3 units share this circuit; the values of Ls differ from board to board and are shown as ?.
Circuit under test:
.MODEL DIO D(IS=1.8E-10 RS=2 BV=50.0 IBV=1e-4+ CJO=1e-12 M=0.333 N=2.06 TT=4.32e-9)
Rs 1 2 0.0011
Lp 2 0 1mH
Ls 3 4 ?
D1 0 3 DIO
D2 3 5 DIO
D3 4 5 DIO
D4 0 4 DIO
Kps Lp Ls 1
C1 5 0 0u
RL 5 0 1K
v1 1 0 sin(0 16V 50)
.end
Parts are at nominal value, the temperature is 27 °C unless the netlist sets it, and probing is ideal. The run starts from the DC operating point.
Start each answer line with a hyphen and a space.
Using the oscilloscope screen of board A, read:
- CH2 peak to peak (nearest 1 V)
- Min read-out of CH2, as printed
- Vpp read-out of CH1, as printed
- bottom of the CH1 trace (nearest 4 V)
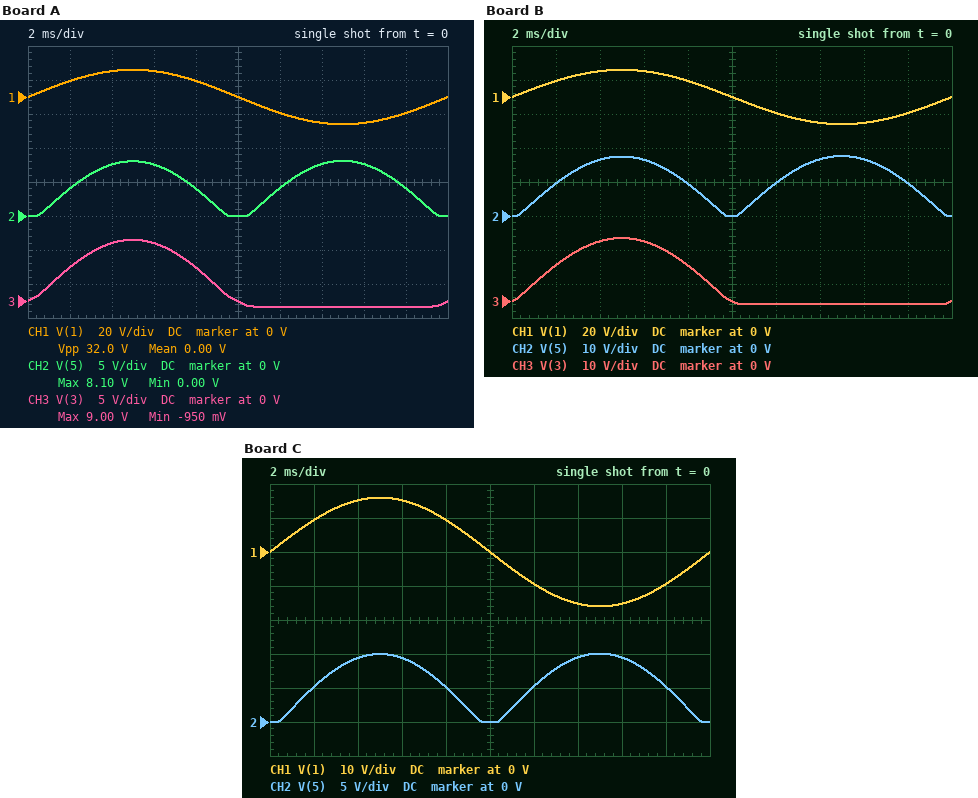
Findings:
- 8 V
- 0.00 V
- 32.0 V
- -16 V
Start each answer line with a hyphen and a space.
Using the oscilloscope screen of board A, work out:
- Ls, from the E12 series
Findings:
- 390 µH
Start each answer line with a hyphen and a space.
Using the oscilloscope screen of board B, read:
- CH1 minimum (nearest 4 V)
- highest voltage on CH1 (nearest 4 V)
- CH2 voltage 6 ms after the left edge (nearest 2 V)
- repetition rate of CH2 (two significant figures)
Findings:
- -16 V
- 16 V
- 16 V
- 100 Hz
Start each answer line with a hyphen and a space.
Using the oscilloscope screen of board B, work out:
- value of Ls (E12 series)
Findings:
- 1.5 mH
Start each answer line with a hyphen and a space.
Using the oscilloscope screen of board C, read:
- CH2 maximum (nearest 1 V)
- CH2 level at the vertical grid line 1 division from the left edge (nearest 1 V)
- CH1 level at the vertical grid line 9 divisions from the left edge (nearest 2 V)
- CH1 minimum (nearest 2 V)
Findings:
- 10 V
- 5 V
- -10 V
- -16 V
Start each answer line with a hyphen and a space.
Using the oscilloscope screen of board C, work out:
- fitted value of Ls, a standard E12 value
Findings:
- 560 µH
